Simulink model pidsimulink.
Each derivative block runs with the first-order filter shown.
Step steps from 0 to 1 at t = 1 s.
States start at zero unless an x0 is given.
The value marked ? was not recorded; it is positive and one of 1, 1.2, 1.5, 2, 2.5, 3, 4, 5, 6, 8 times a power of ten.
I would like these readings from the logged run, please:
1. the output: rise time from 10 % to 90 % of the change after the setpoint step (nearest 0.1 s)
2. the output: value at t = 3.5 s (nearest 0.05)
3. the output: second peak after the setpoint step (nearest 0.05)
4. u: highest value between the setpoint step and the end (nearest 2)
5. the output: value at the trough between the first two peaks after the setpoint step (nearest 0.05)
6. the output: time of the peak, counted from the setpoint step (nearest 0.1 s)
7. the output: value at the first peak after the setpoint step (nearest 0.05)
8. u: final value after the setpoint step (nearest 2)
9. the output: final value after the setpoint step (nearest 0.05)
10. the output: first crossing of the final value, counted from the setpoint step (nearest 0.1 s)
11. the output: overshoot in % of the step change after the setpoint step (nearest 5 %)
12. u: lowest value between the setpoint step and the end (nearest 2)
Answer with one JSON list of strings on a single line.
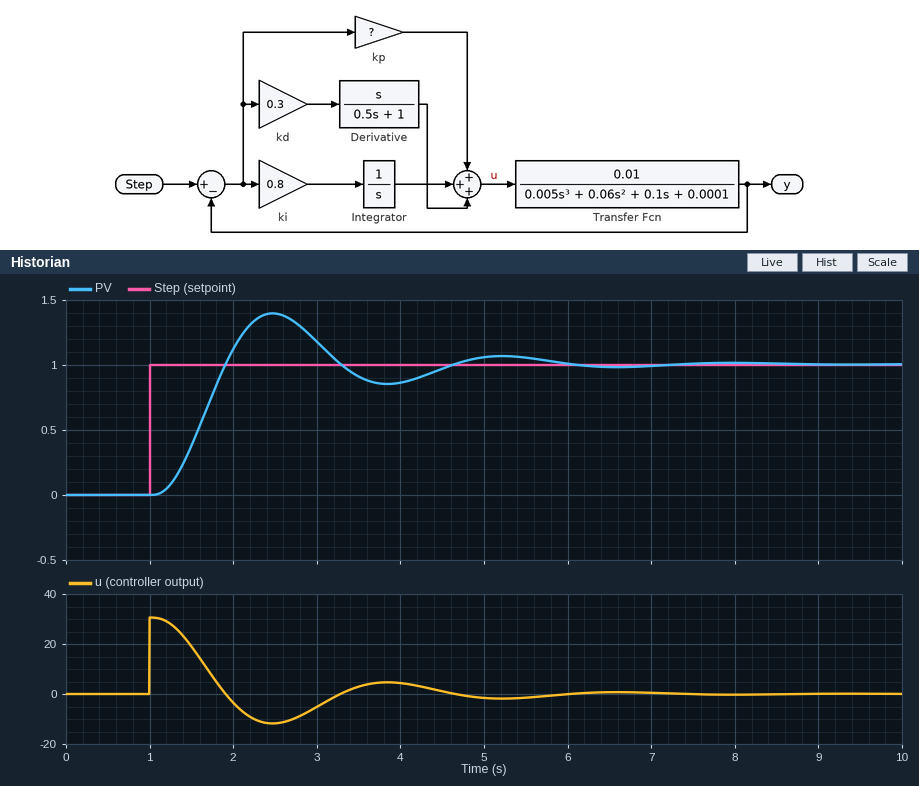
["0.6 s", "0.90", "1.05", "30", "0.85", "1.5 s", "1.40", "0", "1.00", "0.9 s", "40 %", "-12"]
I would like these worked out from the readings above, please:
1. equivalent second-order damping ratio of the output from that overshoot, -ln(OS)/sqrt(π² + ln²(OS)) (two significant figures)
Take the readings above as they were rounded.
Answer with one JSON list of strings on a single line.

["0.28"]
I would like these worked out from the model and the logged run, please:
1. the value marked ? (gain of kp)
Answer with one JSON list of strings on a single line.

["30"]
